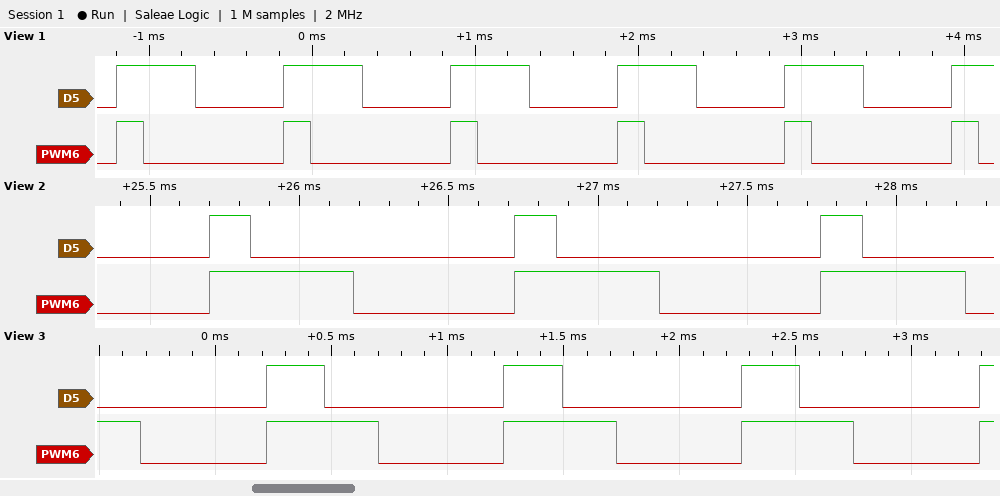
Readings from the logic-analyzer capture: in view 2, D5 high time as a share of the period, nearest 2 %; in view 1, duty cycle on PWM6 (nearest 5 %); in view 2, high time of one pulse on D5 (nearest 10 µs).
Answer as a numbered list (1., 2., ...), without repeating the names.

1. 14 %
2. 15 %
3. 140 µs
